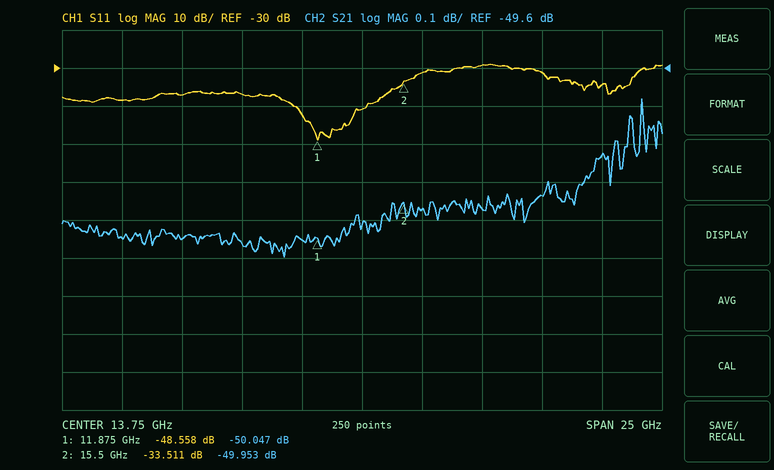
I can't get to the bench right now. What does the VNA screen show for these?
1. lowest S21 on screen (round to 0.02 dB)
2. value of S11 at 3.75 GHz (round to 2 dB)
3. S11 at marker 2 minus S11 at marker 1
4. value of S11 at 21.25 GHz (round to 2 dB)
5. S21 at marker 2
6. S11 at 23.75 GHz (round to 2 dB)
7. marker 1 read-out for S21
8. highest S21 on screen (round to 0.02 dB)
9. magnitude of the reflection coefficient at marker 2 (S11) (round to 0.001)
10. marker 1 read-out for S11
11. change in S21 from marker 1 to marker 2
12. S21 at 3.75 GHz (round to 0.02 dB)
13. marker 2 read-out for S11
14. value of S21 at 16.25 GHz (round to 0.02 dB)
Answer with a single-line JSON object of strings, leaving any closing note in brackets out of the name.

{"lowest S21 on screen": "-50.10 dB", "value of S11 at 3.75 GHz": "-38 dB", "S11 at marker 2 minus S11 at marker 1": "15.047 dB", "value of S11 at 21.25 GHz": "-32 dB", "S21 at marker 2": "-49.953 dB", "S11 at 23.75 GHz": "-34 dB", "marker 1 read-out for S21": "-50.047 dB", "highest S21 on screen": "-49.68 dB", "magnitude of the reflection coefficient at marker 2 (S11)": "0.021", "marker 1 read-out for S11": "-48.558 dB", "change in S21 from marker 1 to marker 2": "0.094 dB", "S21 at 3.75 GHz": "-50.04 dB", "marker 2 read-out for S11": "-33.511 dB", "value of S21 at 16.25 GHz": "-49.98 dB"}
